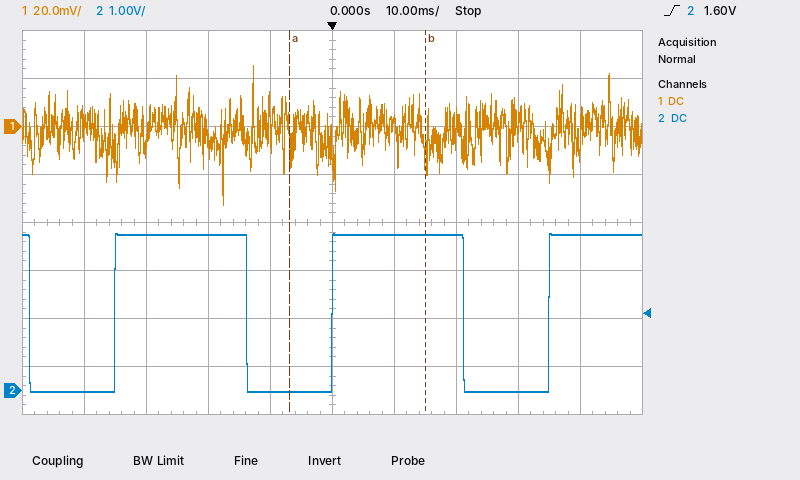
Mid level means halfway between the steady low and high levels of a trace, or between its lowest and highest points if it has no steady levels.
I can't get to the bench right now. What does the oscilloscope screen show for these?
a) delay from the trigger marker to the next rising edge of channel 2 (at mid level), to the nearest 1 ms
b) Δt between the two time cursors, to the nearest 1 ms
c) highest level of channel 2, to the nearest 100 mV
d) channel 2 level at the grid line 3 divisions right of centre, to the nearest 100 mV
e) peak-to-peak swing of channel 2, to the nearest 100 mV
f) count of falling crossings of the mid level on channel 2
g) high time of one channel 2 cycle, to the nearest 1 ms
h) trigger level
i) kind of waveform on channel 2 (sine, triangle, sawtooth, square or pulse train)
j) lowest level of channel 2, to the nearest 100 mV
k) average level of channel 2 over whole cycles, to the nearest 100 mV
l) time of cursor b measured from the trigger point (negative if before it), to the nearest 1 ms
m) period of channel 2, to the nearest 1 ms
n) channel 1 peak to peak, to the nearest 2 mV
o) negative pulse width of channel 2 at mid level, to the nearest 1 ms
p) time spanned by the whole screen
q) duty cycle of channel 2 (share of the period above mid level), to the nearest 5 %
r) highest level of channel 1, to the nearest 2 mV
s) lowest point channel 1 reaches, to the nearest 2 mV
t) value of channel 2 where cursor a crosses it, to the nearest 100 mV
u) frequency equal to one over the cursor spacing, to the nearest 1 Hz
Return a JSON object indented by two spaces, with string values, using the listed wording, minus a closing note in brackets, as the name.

{
  "delay from the trigger marker to the next rising edge of channel 2 (at mid level), to the nearest 1 ms": "35 ms",
  "Δt between the two time cursors, to the nearest 1 ms": "22 ms",
  "highest level of channel 2, to the nearest 100 mV": "3.3 V",
  "channel 2 level at the grid line 3 divisions right of centre, to the nearest 100 mV": "0.0 V",
  "peak-to-peak swing of channel 2, to the nearest 100 mV": "3.3 V",
  "count of falling crossings of the mid level on channel 2": "3",
  "high time of one channel 2 cycle, to the nearest 1 ms": "21 ms",
  "trigger level": "1.60 V",
  "kind of waveform on channel 2": "pulse train",
  "lowest level of channel 2, to the nearest 100 mV": "0.0 V",
  "average level of channel 2 over whole cycles, to the nearest 100 mV": "2.0 V",
  "time of cursor b measured from the trigger point (negative if before it), to the nearest 1 ms": "+15 ms",
  "period of channel 2, to the nearest 1 ms": "35 ms",
  "channel 1 peak to peak, to the nearest 2 mV": "58 mV",
  "negative pulse width of channel 2 at mid level, to the nearest 1 ms": "14 ms",
  "time spanned by the whole screen": "100 ms",
  "duty cycle of channel 2 (share of the period above mid level), to the nearest 5 %": "60 %",
  "highest level of channel 1, to the nearest 2 mV": "26 mV",
  "lowest point channel 1 reaches, to the nearest 2 mV": "-32 mV",
  "value of channel 2 where cursor a crosses it, to the nearest 100 mV": "0.0 V",
  "frequency equal to one over the cursor spacing, to the nearest 1 Hz": "45 Hz"
}
